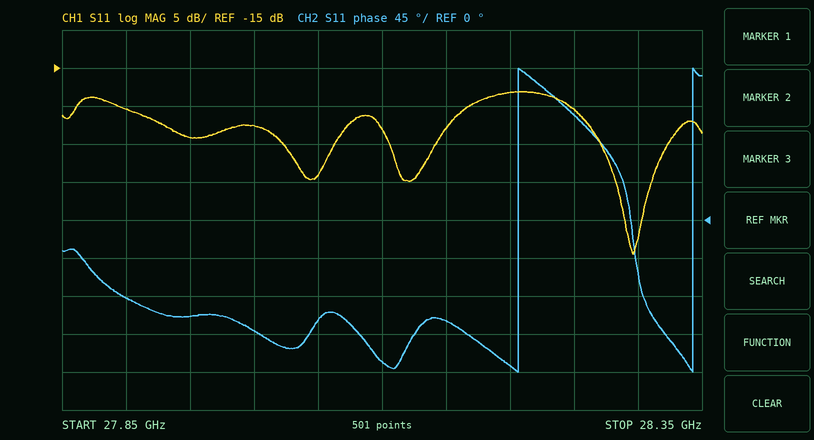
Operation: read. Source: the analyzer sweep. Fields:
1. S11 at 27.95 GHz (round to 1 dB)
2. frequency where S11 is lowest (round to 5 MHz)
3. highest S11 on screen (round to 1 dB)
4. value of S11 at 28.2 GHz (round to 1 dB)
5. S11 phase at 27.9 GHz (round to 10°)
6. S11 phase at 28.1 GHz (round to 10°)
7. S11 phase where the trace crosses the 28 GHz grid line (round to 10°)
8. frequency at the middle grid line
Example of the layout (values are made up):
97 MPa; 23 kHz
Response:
-24 dB; 28.295 GHz; -18 dB; -18 dB; -90°; -170°; -130°; 28.1 GHz
